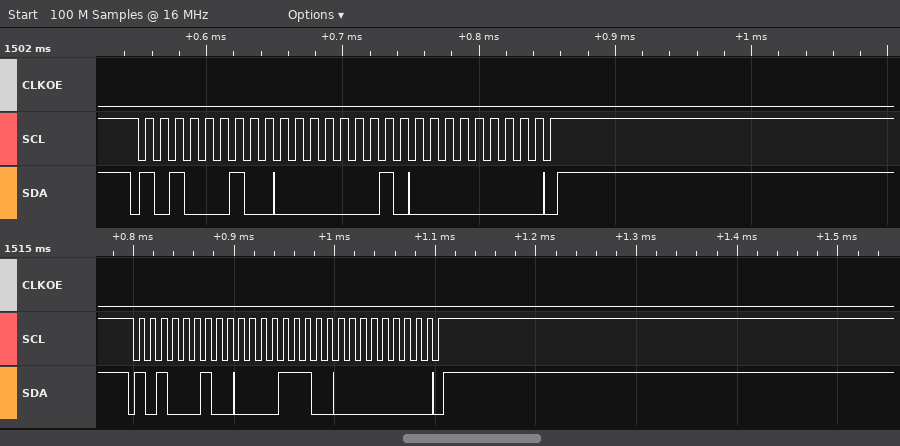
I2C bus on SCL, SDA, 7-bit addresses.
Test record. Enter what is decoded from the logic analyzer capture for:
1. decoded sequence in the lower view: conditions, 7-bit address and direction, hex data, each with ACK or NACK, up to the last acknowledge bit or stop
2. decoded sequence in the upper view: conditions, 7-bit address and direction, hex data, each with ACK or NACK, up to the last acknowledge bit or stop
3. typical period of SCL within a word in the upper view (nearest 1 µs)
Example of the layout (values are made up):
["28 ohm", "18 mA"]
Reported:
["start, address 51 write ACK, 0E ACK, 00 ACK, stop", "start, address 51 write ACK, 01 ACK, 00 ACK, stop", "11 µs"]
